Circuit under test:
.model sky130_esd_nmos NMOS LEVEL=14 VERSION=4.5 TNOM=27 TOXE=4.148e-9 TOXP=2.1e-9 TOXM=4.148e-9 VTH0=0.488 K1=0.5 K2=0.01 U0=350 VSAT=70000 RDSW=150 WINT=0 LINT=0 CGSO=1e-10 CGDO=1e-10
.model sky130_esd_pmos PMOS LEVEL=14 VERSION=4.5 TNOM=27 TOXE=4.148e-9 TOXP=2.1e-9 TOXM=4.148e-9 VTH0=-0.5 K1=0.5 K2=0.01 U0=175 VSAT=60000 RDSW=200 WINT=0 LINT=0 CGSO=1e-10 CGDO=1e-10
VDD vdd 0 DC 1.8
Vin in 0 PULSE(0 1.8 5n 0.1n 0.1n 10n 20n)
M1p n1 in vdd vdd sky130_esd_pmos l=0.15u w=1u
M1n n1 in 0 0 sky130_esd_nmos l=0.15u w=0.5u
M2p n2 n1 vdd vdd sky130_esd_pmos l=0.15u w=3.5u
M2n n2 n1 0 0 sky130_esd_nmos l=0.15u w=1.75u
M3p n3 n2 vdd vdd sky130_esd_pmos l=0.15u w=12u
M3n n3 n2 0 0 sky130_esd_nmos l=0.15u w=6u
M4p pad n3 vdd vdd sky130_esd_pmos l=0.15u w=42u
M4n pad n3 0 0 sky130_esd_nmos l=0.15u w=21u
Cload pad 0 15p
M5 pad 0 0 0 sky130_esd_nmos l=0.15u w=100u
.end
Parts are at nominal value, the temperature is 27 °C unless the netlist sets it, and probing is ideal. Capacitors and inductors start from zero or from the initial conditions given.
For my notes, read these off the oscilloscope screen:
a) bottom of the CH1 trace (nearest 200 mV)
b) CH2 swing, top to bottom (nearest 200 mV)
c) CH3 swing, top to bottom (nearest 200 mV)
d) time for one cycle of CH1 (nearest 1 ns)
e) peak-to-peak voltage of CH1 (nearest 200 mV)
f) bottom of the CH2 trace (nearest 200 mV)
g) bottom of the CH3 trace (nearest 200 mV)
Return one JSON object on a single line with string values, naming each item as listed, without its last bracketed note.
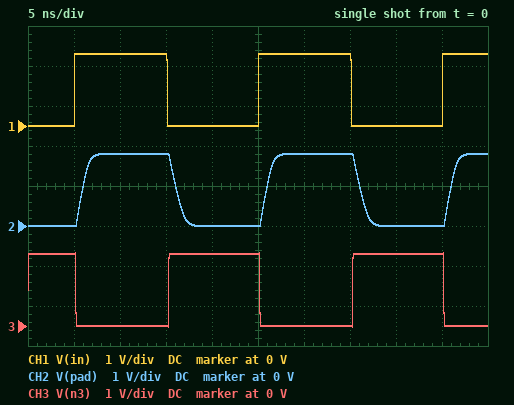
{"bottom of the CH1 trace": "0 V", "CH2 swing, top to bottom": "1.8 V", "CH3 swing, top to bottom": "1.8 V", "time for one cycle of CH1": "20 ns", "peak-to-peak voltage of CH1": "1.8 V", "bottom of the CH2 trace": "0 V", "bottom of the CH3 trace": "0 V"}
